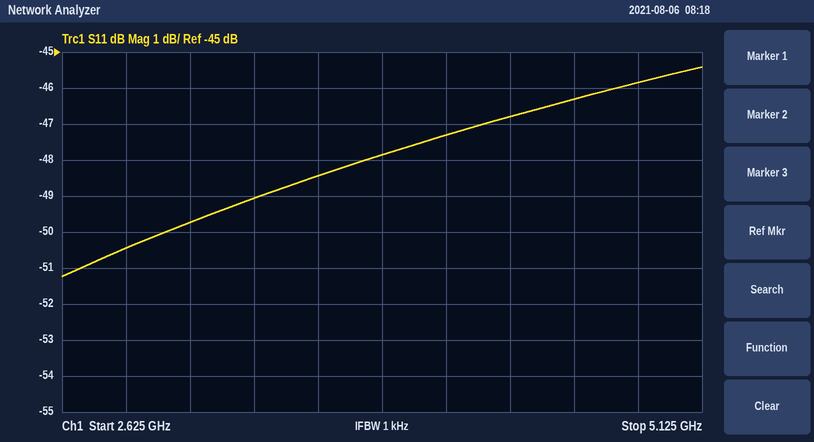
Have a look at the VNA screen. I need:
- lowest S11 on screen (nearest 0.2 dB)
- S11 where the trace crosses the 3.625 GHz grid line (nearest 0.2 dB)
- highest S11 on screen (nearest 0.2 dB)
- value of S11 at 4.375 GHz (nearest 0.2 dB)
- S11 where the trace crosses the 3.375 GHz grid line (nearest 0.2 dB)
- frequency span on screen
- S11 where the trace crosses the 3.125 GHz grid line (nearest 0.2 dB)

-51.2 dB
-48.4 dB
-45.4 dB
-46.8 dB
-49.0 dB
2.5 GHz
-49.8 dB
